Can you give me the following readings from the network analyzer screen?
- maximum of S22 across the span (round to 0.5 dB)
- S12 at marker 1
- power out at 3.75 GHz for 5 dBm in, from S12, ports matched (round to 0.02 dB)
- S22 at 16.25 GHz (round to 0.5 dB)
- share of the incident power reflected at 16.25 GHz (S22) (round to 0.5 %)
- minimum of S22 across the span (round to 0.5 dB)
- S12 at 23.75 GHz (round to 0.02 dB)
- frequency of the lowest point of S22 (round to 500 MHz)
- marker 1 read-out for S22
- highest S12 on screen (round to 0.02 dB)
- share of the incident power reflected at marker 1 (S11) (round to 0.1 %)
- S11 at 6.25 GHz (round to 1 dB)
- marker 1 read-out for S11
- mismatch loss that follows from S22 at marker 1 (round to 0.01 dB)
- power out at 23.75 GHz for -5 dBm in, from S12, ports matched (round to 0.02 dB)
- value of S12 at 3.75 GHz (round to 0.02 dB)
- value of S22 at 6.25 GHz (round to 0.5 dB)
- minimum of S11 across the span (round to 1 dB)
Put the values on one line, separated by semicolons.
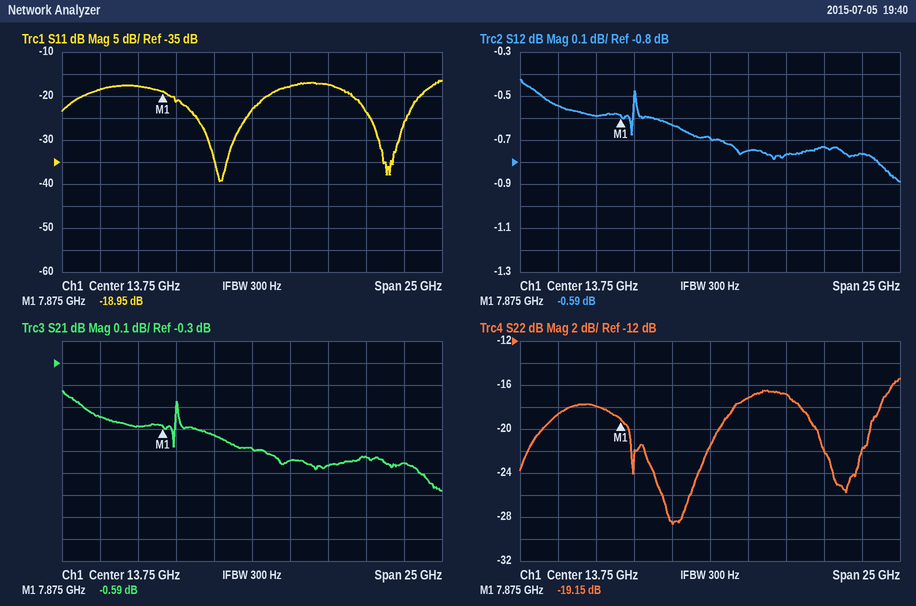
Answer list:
-15.5 dB; -0.59 dB; 4.46 dBm; -17.0 dB; 2.0 %; -28.5 dB; -0.76 dB; 11.5 GHz; -19.15 dB; -0.42 dB; 1.3 %; -18 dB; -18.95 dB; 0.05 dB; -5.76 dBm; -0.54 dB; -18.0 dB; -39 dB
